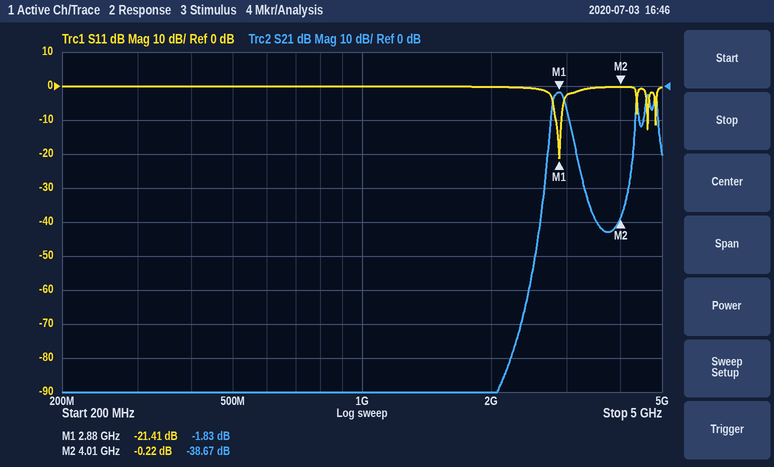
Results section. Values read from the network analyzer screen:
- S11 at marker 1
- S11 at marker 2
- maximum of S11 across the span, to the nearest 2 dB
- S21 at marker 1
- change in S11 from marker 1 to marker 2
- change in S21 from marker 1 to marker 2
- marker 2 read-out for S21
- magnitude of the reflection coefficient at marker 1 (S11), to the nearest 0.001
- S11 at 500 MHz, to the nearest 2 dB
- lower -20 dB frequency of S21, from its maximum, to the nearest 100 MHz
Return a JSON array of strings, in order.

["-21.41 dB", "-0.22 dB", "0 dB", "-1.83 dB", "21.19 dB", "-36.84 dB", "-38.67 dB", "0.085", "0 dB", "2.7 GHz"]
